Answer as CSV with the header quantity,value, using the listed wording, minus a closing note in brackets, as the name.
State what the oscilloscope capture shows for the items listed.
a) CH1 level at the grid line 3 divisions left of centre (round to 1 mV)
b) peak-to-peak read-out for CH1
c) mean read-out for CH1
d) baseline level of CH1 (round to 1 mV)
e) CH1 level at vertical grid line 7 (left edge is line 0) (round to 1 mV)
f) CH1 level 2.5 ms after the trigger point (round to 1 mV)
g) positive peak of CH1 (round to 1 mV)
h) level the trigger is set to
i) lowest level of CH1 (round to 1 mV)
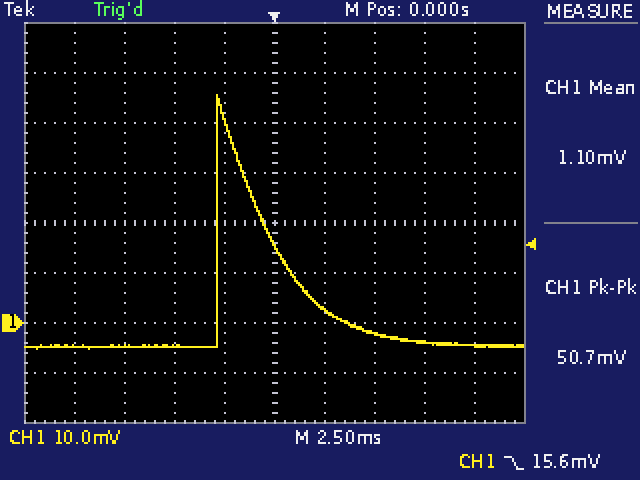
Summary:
quantity,value
CH1 level at the grid line 3 divisions left of centre,-5 mV
peak-to-peak read-out for CH1,50.7 mV
mean read-out for CH1,1.10 mV
baseline level of CH1,-5 mV
CH1 level at vertical grid line 7 (left edge is line 0),-2 mV
CH1 level 2.5 ms after the trigger point,3 mV
positive peak of CH1,46 mV
level the trigger is set to,15.6 mV
lowest level of CH1,-5 mV
